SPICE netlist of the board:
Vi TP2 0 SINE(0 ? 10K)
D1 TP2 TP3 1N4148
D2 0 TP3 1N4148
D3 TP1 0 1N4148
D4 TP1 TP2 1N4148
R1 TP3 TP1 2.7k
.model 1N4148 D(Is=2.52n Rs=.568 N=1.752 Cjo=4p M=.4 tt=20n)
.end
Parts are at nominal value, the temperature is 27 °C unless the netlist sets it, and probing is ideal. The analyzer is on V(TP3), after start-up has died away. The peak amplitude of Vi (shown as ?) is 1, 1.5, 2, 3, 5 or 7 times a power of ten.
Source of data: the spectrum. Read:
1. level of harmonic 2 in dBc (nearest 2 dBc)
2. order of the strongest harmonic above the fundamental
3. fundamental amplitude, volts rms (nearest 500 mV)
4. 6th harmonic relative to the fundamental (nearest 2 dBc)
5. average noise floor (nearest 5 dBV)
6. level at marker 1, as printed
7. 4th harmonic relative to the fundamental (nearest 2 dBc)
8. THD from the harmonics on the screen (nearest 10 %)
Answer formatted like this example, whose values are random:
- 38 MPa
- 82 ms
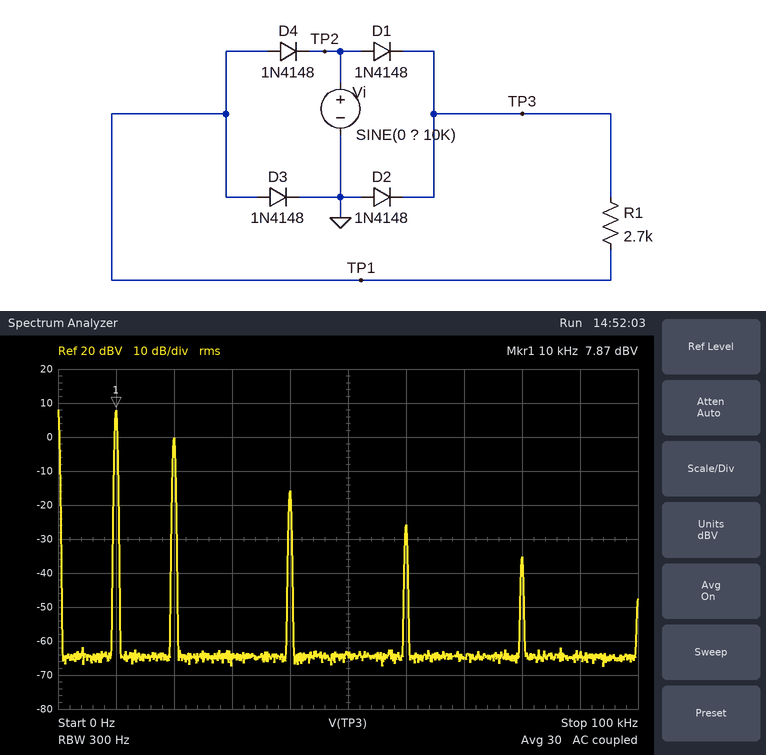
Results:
- -8 dBc
- 2
- 2.5 V
- -34 dBc
- -65 dBV
- 7.87 dBV
- -24 dBc
- 40 %
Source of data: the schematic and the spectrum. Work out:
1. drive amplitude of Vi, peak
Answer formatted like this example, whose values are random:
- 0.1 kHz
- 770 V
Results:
- 7 V
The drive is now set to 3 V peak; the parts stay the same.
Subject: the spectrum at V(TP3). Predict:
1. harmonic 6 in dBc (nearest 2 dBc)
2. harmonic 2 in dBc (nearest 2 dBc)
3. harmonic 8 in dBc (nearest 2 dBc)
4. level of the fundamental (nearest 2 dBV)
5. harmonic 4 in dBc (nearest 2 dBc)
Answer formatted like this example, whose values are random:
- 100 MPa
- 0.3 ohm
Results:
- -42 dBc
- -10 dBc
- -40 dBc
- 0 dBV
- -34 dBc
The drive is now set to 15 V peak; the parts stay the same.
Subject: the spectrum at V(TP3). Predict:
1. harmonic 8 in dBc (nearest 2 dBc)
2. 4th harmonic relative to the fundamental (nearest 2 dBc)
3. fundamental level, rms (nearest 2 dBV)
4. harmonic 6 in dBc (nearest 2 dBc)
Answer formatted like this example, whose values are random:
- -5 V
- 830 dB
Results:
- -36 dBc
- -22 dBc
- 14 dBV
- -30 dBc
